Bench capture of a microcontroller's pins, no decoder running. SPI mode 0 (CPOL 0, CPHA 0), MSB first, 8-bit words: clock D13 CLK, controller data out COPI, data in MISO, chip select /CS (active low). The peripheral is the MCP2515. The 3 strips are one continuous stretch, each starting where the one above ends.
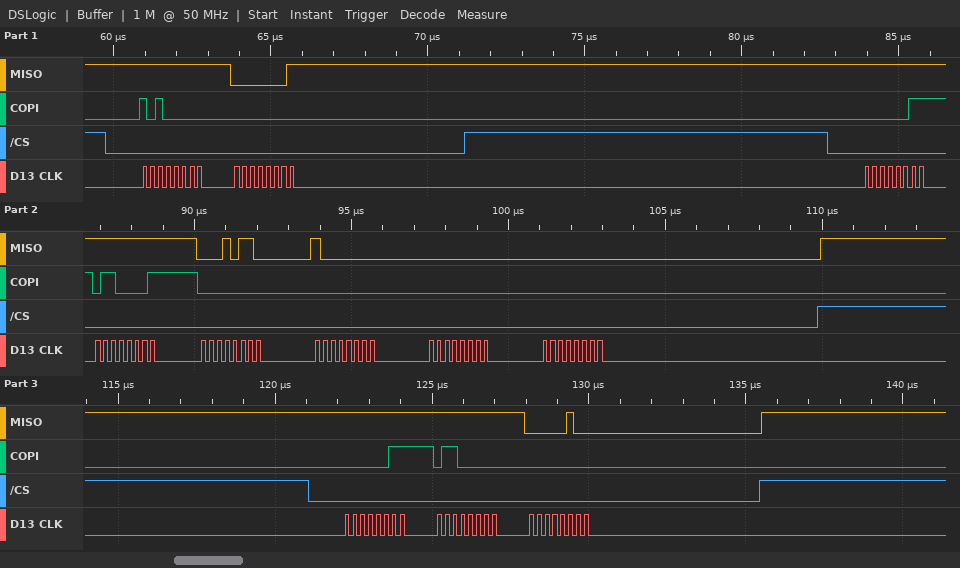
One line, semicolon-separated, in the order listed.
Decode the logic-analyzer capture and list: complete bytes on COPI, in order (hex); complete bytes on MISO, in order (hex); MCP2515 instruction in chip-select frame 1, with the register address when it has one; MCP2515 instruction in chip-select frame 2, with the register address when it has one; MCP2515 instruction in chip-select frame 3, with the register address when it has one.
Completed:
A0 00 03 61 00 00 00 00 03 60 00; FF 01 FF FF 16 80 00 00 FF FF 04; READ STATUS; READ 0x61; READ 0x60
